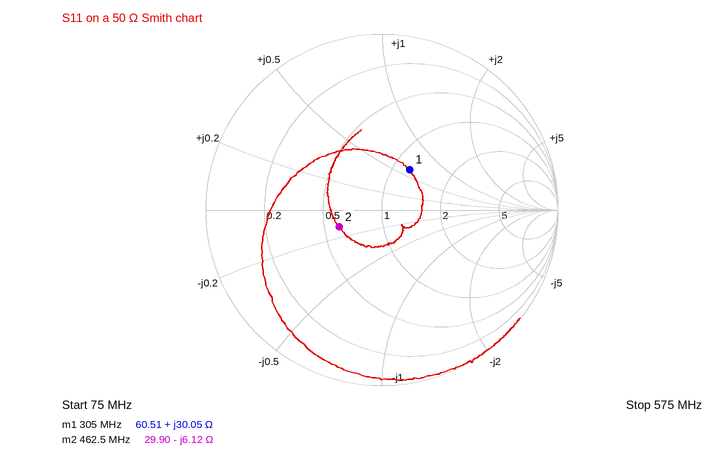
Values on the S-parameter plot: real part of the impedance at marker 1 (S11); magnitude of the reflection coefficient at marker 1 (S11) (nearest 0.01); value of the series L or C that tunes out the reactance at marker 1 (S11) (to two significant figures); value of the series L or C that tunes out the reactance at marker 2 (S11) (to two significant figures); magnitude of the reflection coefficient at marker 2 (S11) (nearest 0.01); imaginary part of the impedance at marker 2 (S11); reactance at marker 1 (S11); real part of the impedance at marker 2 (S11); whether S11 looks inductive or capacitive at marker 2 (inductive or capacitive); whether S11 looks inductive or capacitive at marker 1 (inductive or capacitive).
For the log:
60.51 Ω
0.28
17 pF
2.1 nH
0.26
-6.12 Ω
+30.05 Ω
29.90 Ω
capacitive
inductive
